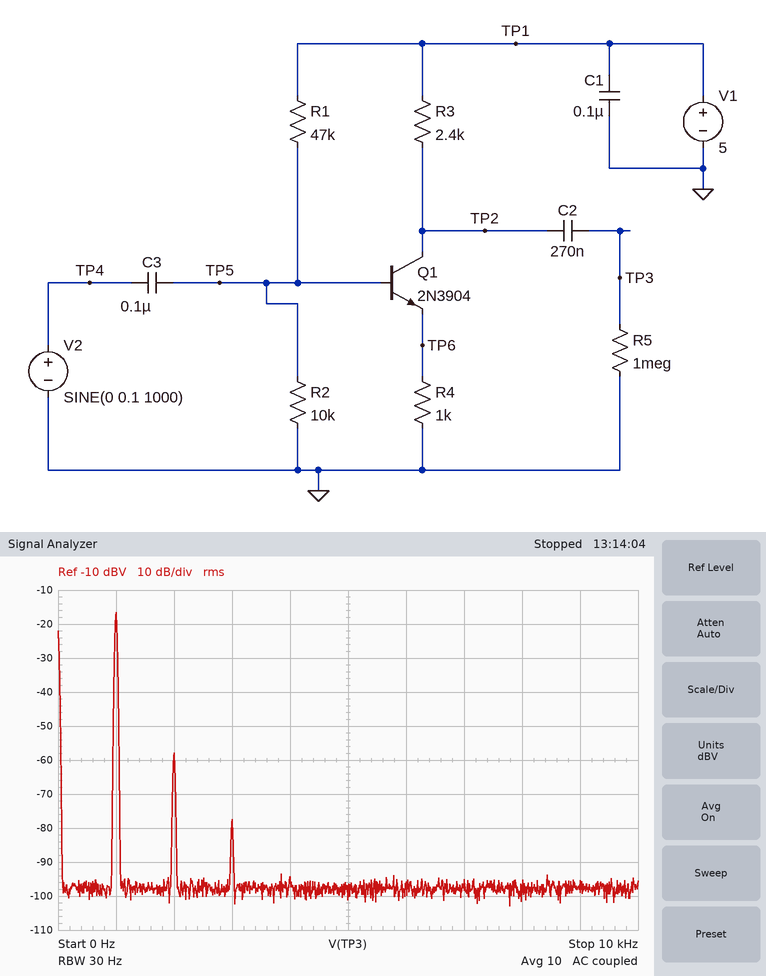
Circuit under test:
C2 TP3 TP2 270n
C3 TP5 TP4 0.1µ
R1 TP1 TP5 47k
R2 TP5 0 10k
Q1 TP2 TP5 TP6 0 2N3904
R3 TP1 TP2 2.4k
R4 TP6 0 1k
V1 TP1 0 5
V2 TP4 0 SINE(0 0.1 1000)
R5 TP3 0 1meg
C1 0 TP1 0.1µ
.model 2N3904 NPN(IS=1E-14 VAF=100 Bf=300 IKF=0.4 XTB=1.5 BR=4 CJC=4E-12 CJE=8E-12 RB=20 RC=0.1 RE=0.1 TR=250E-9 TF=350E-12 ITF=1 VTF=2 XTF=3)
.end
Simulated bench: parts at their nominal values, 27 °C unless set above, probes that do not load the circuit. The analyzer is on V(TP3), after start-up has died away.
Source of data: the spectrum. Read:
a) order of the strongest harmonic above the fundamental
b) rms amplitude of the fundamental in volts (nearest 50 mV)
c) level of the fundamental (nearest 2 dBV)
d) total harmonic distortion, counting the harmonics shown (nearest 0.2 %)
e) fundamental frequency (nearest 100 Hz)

2
150 mV
-16 dBV
0.8 %
1.0 kHz
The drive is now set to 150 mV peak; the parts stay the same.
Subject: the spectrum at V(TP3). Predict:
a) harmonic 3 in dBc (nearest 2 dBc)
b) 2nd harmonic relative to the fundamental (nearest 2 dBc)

-54 dBc
-38 dBc
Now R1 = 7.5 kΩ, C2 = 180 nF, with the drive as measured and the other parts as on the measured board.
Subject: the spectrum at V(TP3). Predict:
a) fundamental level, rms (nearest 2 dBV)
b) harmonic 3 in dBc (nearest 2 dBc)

-34 dBV
-52 dBc
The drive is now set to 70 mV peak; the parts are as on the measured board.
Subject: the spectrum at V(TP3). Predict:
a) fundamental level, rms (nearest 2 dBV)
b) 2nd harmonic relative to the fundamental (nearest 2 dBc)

-20 dBV
-44 dBc
